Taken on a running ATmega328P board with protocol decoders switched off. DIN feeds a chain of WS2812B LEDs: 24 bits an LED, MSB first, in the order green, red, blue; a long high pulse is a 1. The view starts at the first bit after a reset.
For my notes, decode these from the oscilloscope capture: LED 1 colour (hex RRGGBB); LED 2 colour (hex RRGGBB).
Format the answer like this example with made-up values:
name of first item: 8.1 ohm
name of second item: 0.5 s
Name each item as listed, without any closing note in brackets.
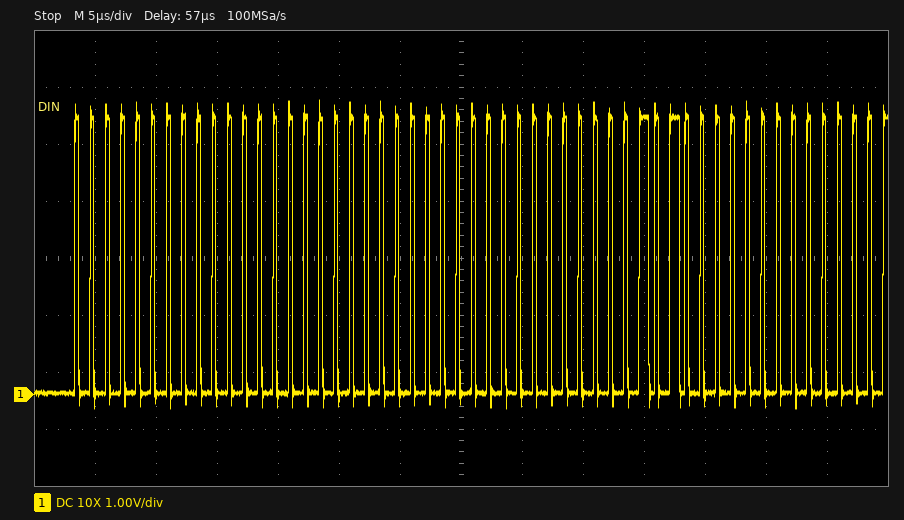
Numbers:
LED 1 colour: #000000
LED 2 colour: #050000
